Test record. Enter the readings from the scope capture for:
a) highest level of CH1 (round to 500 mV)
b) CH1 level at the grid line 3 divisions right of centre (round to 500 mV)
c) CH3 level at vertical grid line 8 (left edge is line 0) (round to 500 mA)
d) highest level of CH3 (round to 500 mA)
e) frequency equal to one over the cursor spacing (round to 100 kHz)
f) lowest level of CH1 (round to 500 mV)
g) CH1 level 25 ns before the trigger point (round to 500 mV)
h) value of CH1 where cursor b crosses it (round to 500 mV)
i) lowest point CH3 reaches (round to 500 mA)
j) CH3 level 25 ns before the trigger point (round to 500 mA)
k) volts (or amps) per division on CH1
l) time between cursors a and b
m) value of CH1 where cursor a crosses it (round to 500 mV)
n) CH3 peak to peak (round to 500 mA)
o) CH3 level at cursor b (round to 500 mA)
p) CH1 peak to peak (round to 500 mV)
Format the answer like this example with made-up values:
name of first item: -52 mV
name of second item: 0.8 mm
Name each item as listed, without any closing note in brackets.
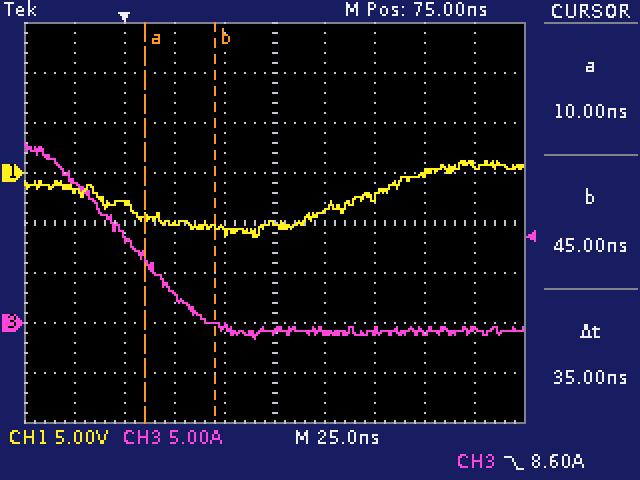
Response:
highest level of CH1: 1.0 V
CH1 level at the grid line 3 divisions right of centre: 0.0 V
CH3 level at vertical grid line 8 (left edge is line 0): -1.0 A
highest level of CH3: 18.0 A
frequency equal to one over the cursor spacing: 28.6 MHz
lowest level of CH1: -6.5 V
CH1 level 25 ns before the trigger point: -1.5 V
value of CH1 where cursor b crosses it: -5.5 V
lowest point CH3 reaches: -1.5 A
CH3 level 25 ns before the trigger point: 14.0 A
volts (or amps) per division on CH1: 5 V
time between cursors a and b: 35 ns
value of CH1 where cursor a crosses it: -4.5 V
CH3 peak to peak: 19.5 A
CH3 level at cursor b: -500 mA
CH1 peak to peak: 7.5 V
